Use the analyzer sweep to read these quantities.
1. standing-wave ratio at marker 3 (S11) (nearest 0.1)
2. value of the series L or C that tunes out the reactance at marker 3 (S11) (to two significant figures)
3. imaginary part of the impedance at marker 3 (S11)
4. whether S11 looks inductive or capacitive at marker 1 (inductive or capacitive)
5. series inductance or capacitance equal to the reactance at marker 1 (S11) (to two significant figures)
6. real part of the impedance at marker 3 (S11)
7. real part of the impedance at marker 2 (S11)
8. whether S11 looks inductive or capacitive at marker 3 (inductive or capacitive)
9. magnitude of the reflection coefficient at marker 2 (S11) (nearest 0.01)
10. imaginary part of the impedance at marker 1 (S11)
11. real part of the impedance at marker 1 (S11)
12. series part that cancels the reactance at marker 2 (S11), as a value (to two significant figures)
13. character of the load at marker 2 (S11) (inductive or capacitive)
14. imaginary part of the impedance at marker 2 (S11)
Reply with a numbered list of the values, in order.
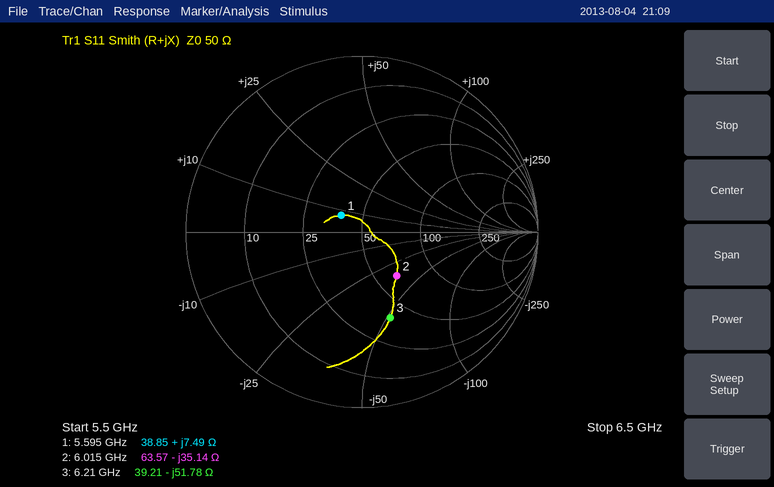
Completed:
1. 3.1
2. 1.3 nH
3. -51.78 Ω
4. inductive
5. 210 pH
6. 39.21 Ω
7. 63.57 Ω
8. capacitive
9. 0.32
10. +7.49 Ω
11. 38.85 Ω
12. 930 pH
13. capacitive
14. -35.14 Ω
